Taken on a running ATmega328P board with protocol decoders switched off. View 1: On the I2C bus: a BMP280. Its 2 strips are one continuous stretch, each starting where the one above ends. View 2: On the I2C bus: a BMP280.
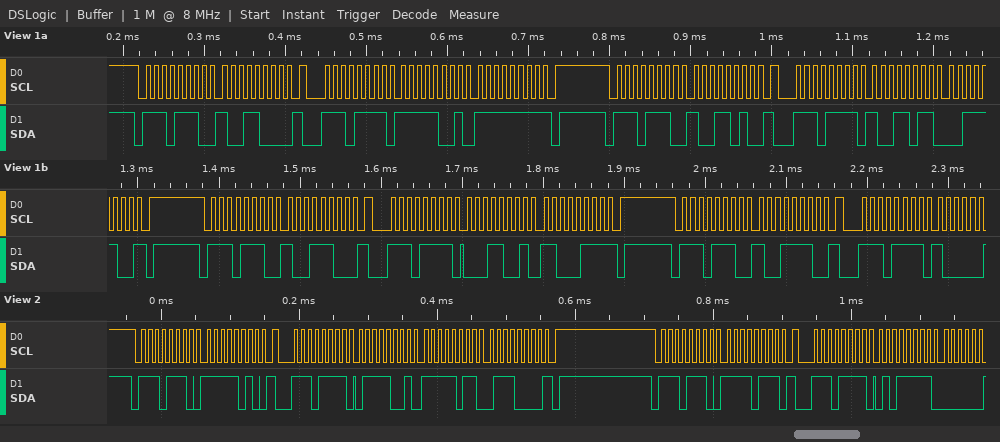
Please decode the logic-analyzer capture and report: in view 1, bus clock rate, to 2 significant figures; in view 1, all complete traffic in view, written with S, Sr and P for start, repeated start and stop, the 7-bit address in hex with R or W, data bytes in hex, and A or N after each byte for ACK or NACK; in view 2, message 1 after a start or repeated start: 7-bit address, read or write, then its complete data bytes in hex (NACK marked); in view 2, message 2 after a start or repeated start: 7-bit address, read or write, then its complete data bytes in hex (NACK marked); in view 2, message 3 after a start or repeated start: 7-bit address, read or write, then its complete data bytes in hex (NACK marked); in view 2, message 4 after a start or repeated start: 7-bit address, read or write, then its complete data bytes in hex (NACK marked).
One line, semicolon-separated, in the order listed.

100 kHz; S 77W A 98 A Sr 77R A F9 A FF N P S 77W A 9A A Sr 77R A 9B A 3C N P S 77W A 9C A Sr 77R A 19 A C7 N P S 77W A 9E A Sr 77R A; 0x77 write: FA; 0x77 read: 79 FB 70 NACK; 0x77 write: F7; 0x77 read: 5F
